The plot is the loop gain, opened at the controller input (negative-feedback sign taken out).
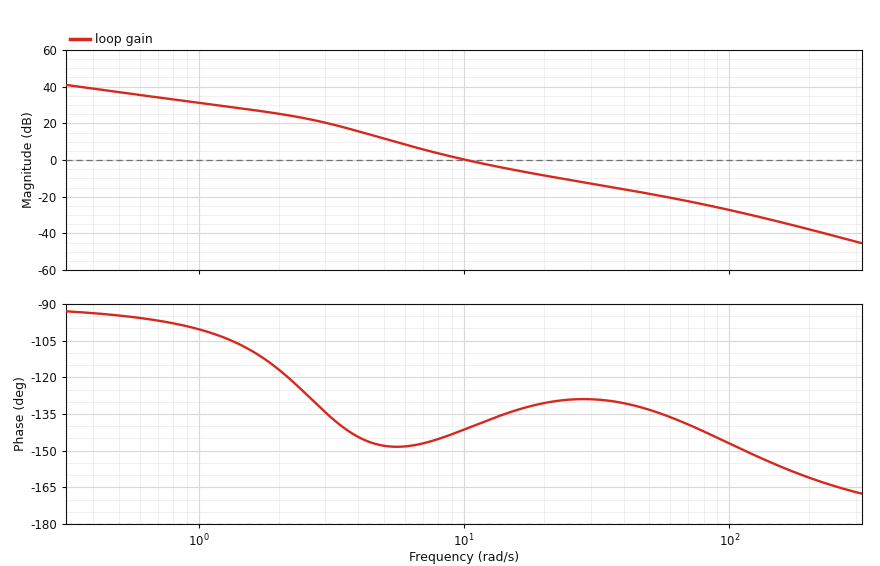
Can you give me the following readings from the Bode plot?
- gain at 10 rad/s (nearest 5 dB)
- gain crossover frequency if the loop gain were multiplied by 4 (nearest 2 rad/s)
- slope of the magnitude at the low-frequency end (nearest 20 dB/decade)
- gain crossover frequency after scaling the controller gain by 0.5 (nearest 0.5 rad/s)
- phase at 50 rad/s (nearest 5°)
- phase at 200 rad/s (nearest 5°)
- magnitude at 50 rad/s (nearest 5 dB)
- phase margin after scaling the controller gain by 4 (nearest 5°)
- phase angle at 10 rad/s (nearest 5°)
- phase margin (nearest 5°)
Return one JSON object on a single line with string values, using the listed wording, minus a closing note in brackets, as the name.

{"gain at 10 rad/s": "0 dB", "gain crossover frequency if the loop gain were multiplied by 4": "28 rad/s", "slope of the magnitude at the low-frequency end": "-20 dB/decade", "gain crossover frequency after scaling the controller gain by 0.5": "7.0 rad/s", "phase at 50 rad/s": "-135°", "phase at 200 rad/s": "-160°", "magnitude at 50 rad/s": "-20 dB", "phase margin after scaling the controller gain by 4": "50°", "phase angle at 10 rad/s": "-140°", "phase margin": "40°"}
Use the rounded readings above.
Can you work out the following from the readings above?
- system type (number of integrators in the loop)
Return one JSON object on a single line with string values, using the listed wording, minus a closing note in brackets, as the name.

{"system type": "1"}
